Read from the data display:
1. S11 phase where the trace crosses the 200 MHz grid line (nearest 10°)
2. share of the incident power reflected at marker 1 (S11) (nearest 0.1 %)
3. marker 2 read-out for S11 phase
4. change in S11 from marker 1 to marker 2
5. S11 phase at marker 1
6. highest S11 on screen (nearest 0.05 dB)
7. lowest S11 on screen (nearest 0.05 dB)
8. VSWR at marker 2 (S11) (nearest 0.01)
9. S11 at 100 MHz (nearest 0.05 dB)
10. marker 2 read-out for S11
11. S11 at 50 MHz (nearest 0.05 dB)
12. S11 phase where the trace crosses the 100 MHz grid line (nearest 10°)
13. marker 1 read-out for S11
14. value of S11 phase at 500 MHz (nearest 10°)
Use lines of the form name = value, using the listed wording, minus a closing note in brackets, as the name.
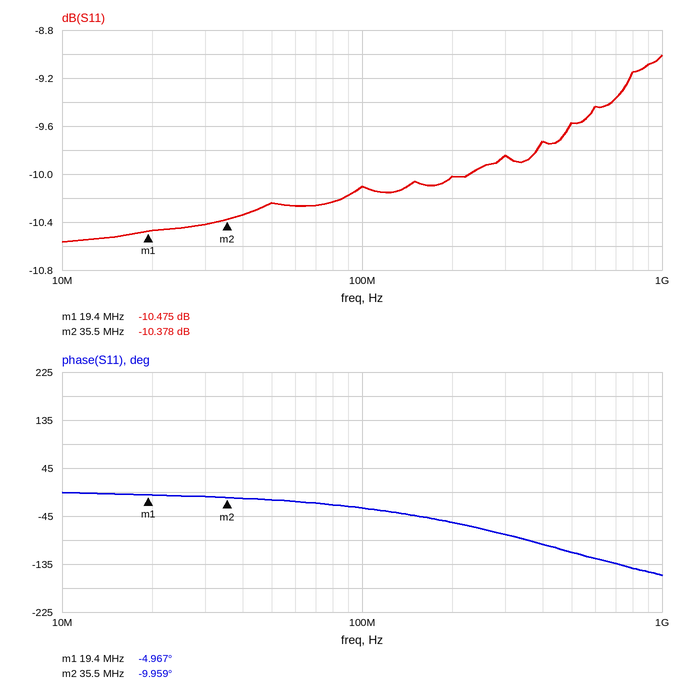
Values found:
S11 phase where the trace crosses the 200 MHz grid line = -60°
share of the incident power reflected at marker 1 (S11) = 9.0 %
marker 2 read-out for S11 phase = -9.959°
change in S11 from marker 1 to marker 2 = 0.097 dB
S11 phase at marker 1 = -4.967°
highest S11 on screen = -9.00 dB
lowest S11 on screen = -10.55 dB
VSWR at marker 2 (S11) = 1.87
S11 at 100 MHz = -10.10 dB
marker 2 read-out for S11 = -10.378 dB
S11 at 50 MHz = -10.25 dB
S11 phase where the trace crosses the 100 MHz grid line = -30°
marker 1 read-out for S11 = -10.475 dB
value of S11 phase at 500 MHz = -110°
